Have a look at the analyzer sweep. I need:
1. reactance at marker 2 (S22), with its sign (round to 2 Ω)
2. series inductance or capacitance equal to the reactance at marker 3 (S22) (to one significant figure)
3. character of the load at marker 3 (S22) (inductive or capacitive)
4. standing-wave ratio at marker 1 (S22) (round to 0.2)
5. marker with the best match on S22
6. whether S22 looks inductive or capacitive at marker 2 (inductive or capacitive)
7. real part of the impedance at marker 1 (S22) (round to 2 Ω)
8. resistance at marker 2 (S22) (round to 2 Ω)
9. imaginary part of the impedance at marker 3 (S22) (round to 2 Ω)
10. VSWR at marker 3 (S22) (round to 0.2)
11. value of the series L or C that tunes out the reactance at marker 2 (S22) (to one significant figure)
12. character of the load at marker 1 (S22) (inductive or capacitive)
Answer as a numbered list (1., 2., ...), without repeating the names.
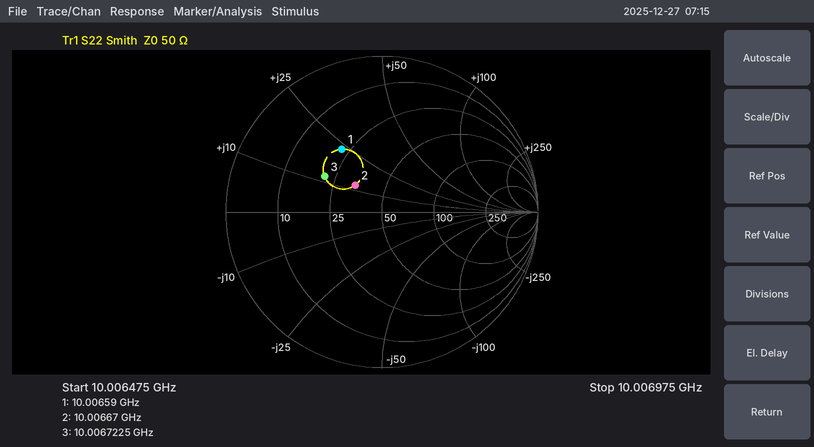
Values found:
1. +12 Ω
2. 200 pH
3. inductive
4. 2.8
5. marker 2
6. inductive
7. 22 Ω
8. 34 Ω
9. +12 Ω
10. 2.6
11. 1 pF
12. inductive
